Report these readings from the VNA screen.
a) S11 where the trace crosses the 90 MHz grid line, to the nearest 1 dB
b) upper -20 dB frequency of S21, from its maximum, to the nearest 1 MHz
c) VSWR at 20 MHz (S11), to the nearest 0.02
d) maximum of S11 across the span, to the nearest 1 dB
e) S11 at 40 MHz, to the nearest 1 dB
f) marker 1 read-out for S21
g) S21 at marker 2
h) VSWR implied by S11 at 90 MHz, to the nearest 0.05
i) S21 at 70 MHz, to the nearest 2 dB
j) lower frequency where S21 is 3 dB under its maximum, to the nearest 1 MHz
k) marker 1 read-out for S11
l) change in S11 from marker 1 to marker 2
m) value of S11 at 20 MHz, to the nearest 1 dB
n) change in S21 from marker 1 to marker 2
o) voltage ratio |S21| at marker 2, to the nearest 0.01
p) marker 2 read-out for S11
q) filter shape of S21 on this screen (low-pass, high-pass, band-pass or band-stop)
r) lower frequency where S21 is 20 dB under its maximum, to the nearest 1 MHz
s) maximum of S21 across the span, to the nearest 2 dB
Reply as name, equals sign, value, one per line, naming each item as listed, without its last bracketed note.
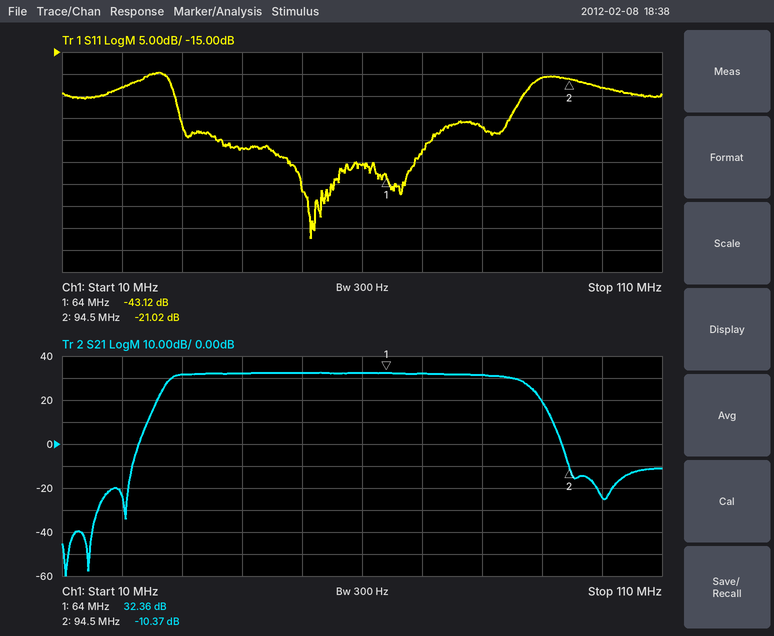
S11 where the trace crosses the 90 MHz grid line, to the nearest 1 dB = -21 dB
upper -20 dB frequency of S21, from its maximum, to the nearest 1 MHz = 91 MHz
VSWR at 20 MHz (S11), to the nearest 0.02 = 1.16
maximum of S11 across the span, to the nearest 1 dB = -20 dB
S11 at 40 MHz, to the nearest 1 dB = -37 dB
marker 1 read-out for S21 = 32.36 dB
S21 at marker 2 = -10.37 dB
VSWR implied by S11 at 90 MHz, to the nearest 0.05 = 1.20
S21 at 70 MHz, to the nearest 2 dB = 32 dB
lower frequency where S21 is 3 dB under its maximum, to the nearest 1 MHz = 28 MHz
marker 1 read-out for S11 = -43.12 dB
change in S11 from marker 1 to marker 2 = 22.10 dB
value of S11 at 20 MHz, to the nearest 1 dB = -23 dB
change in S21 from marker 1 to marker 2 = -42.73 dB
voltage ratio |S21| at marker 2, to the nearest 0.01 = 0.30
marker 2 read-out for S11 = -21.02 dB
filter shape of S21 on this screen = band-pass
lower frequency where S21 is 20 dB under its maximum, to the nearest 1 MHz = 25 MHz
maximum of S21 across the span, to the nearest 2 dB = 32 dB
